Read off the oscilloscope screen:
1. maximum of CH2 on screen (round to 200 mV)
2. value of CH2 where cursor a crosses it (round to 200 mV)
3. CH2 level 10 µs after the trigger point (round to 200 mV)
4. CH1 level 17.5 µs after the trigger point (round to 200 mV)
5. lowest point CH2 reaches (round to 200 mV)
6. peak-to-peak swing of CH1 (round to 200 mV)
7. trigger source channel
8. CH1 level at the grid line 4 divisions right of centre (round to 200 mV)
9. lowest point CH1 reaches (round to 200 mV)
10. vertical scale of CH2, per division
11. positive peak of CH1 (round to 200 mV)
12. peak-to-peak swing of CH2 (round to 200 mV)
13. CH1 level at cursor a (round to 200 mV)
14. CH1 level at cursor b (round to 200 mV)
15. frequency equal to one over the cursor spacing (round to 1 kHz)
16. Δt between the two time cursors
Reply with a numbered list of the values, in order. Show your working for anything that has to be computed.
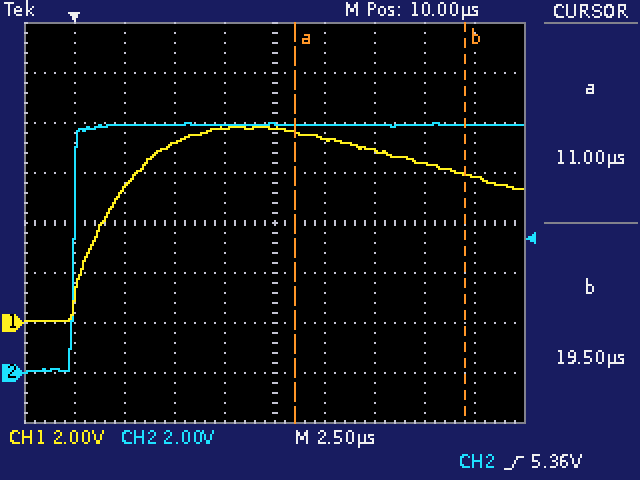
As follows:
1. 10.0 V
2. 10.0 V
3. 10.0 V
4. 6.4 V
5. 0.0 V
6. 7.8 V − (0.0 V) = 7.8 V
7. CH2
8. 5.8 V
9. 0.0 V
10. 2 V
11. 7.8 V
12. 10.0 V − (0.0 V) = 10.0 V
13. 7.6 V
14. 6.0 V
15. 1 / 8.50 µs ≈ 118 kHz
16. 19.5 µs − (11 µs) = 8.50 µs
